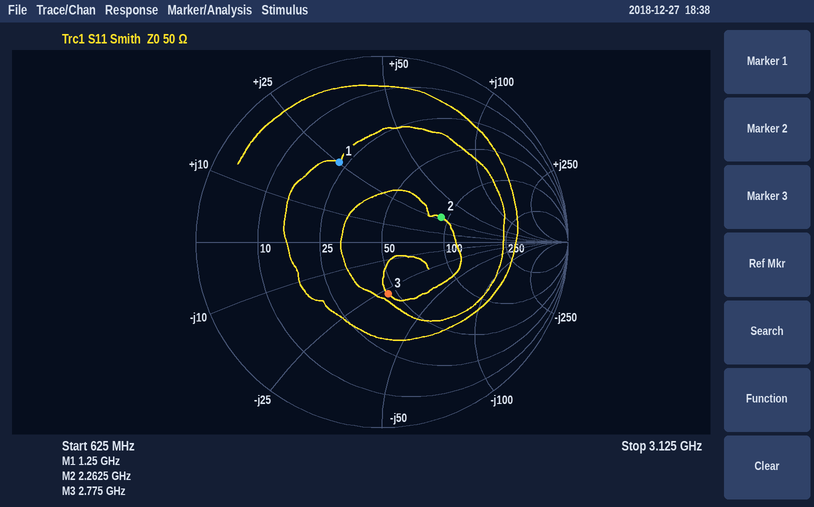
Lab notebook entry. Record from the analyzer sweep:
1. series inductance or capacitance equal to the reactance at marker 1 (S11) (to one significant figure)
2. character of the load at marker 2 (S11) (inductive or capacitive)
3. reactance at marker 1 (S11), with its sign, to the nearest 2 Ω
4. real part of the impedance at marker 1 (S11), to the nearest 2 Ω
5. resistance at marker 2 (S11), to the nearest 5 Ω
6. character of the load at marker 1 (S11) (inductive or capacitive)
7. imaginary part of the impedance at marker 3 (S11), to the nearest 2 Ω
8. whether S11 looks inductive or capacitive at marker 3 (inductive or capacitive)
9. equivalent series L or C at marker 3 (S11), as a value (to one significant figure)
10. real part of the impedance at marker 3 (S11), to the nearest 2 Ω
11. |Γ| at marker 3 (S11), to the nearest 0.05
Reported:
3 nH
inductive
+26 Ω
22 Ω
90 Ω
inductive
-28 Ω
capacitive
2 pF
46 Ω
0.30
